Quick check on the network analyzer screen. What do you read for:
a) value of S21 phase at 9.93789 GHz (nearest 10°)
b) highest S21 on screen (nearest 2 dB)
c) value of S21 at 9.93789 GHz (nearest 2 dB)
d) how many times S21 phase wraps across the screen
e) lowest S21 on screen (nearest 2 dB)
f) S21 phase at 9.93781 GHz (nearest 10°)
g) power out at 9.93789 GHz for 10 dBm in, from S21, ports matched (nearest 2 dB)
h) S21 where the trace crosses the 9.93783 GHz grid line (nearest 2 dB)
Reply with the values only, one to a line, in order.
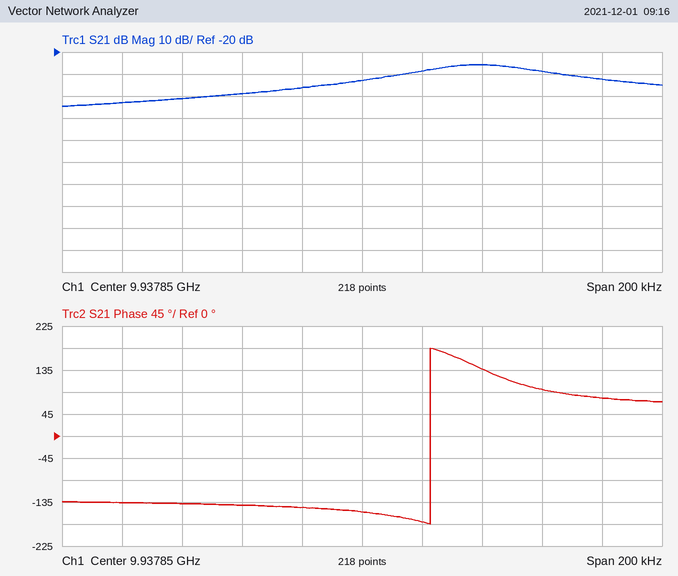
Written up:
140°
-26 dB
-26 dB
1
-44 dB
-140°
-16 dBm
-36 dB
